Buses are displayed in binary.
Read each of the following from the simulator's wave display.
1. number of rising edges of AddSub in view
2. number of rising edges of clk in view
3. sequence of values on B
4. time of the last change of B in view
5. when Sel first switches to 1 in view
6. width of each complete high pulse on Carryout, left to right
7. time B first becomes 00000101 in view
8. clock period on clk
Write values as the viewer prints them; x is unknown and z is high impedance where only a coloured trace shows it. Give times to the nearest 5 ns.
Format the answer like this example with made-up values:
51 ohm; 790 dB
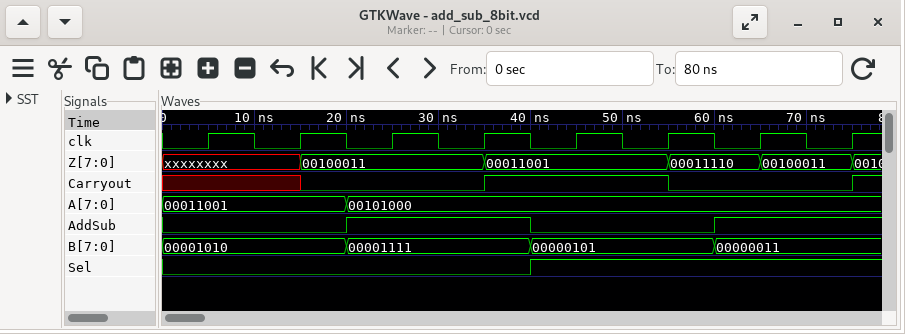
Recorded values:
2; 8; 00001010, 00001111, 00000101, 00000011; 60 ns; 40 ns; 20 ns; 40 ns; 10 ns
